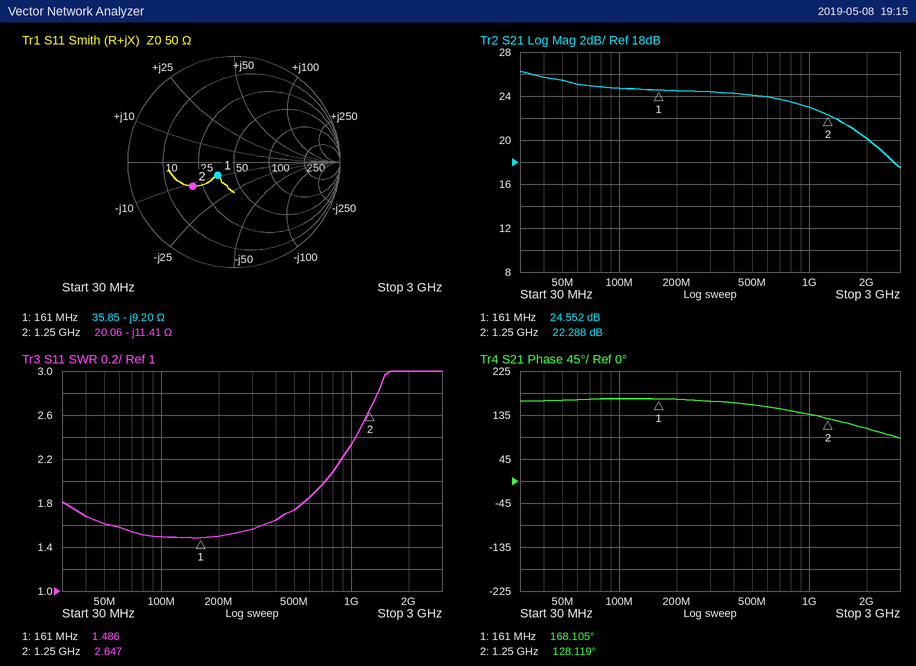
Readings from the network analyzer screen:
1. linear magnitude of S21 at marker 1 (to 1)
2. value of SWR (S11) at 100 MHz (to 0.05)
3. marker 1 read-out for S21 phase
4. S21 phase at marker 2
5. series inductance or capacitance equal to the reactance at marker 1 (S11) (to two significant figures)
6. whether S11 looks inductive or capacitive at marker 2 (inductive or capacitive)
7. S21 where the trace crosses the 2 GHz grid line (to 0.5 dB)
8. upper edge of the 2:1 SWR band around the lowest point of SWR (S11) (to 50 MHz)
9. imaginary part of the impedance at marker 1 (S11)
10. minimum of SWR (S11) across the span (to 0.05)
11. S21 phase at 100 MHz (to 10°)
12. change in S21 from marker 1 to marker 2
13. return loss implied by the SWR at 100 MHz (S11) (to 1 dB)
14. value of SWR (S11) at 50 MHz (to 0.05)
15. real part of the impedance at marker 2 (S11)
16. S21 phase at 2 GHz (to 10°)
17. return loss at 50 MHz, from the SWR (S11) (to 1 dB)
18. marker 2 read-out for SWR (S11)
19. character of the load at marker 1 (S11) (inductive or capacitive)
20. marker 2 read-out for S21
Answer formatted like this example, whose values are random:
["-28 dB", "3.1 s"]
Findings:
["17", "1.50", "168.105°", "128.119°", "110 pF", "capacitive", "20.0 dB", "750 MHz", "-9.20 Ω", "1.50", "170°", "-2.264 dB", "14 dB", "1.60", "20.06 Ω", "110°", "13 dB", "2.647", "capacitive", "22.288 dB"]
